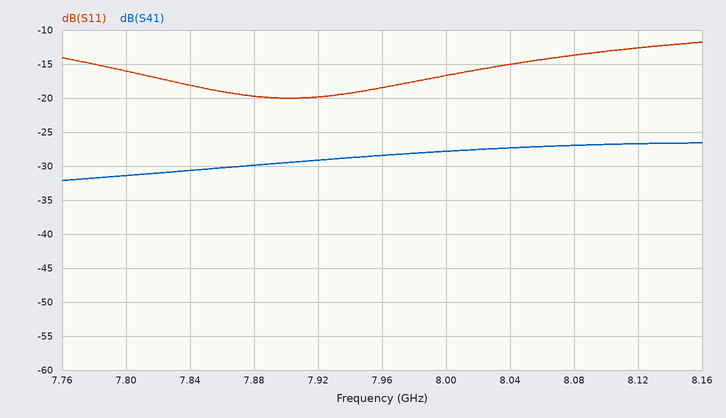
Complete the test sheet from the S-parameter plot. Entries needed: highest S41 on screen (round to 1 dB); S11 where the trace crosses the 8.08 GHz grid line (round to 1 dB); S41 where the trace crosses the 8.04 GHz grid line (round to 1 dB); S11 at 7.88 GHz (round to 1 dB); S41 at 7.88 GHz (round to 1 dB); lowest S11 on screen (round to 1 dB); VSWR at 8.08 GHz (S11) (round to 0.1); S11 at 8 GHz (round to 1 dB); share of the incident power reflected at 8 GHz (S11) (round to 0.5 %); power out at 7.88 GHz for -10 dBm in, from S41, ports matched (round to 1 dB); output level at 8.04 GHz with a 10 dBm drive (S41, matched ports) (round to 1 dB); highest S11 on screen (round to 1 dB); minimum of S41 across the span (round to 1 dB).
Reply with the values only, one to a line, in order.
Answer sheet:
-27 dB
-14 dB
-27 dB
-20 dB
-30 dB
-20 dB
1.5
-17 dB
2.0 %
-40 dBm
-17 dBm
-12 dB
-32 dB
